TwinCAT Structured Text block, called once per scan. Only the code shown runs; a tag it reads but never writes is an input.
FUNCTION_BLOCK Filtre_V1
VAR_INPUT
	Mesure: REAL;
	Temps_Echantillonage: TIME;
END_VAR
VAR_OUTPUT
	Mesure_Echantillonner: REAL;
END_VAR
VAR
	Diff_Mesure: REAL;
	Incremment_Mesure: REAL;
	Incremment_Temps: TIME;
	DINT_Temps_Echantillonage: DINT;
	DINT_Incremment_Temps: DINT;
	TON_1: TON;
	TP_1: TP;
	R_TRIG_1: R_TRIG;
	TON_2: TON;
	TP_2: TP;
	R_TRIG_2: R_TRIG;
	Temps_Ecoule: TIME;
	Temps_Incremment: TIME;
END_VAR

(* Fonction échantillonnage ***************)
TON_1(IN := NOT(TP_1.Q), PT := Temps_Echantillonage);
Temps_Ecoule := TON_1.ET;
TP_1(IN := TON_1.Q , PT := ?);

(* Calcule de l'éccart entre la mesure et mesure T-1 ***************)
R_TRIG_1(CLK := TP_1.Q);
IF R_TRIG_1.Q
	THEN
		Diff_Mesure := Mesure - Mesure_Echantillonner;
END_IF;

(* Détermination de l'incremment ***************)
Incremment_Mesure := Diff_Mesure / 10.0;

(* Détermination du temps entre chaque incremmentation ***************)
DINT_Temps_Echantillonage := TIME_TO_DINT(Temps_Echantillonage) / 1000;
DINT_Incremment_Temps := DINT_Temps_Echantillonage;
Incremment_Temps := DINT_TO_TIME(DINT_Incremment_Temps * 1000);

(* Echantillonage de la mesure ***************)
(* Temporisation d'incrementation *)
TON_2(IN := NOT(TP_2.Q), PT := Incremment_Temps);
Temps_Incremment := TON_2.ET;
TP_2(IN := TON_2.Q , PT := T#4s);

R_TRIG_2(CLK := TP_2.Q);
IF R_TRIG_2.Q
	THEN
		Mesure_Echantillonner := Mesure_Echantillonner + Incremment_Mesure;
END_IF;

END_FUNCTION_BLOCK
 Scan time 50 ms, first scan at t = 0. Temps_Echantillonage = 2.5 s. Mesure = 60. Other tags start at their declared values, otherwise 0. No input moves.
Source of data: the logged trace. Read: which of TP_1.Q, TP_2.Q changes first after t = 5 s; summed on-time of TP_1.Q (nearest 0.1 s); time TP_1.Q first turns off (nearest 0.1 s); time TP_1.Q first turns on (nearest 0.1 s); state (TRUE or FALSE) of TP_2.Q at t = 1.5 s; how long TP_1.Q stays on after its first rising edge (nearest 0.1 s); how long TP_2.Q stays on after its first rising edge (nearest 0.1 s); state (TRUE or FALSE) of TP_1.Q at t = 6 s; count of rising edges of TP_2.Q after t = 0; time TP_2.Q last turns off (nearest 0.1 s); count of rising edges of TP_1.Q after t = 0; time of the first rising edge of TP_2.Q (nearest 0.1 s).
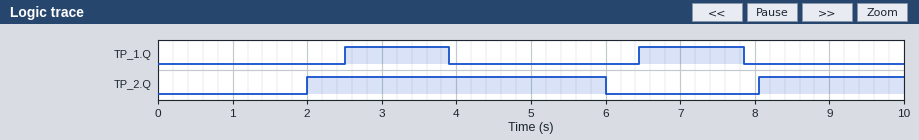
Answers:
TP_2.Q
2.8 s
3.9 s
2.5 s
FALSE
1.4 s
4.0 s
FALSE
2
6.0 s
2
2.0 s
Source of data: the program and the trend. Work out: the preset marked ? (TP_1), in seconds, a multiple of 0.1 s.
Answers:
1.4 s
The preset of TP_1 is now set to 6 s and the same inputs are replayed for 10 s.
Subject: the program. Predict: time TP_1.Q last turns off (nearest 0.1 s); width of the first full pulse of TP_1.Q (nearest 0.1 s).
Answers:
8.5 s
6.0 s
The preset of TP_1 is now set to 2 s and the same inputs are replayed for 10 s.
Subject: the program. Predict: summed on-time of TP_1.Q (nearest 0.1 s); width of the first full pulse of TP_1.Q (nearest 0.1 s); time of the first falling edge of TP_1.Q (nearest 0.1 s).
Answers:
4.0 s
2.0 s
4.5 s
